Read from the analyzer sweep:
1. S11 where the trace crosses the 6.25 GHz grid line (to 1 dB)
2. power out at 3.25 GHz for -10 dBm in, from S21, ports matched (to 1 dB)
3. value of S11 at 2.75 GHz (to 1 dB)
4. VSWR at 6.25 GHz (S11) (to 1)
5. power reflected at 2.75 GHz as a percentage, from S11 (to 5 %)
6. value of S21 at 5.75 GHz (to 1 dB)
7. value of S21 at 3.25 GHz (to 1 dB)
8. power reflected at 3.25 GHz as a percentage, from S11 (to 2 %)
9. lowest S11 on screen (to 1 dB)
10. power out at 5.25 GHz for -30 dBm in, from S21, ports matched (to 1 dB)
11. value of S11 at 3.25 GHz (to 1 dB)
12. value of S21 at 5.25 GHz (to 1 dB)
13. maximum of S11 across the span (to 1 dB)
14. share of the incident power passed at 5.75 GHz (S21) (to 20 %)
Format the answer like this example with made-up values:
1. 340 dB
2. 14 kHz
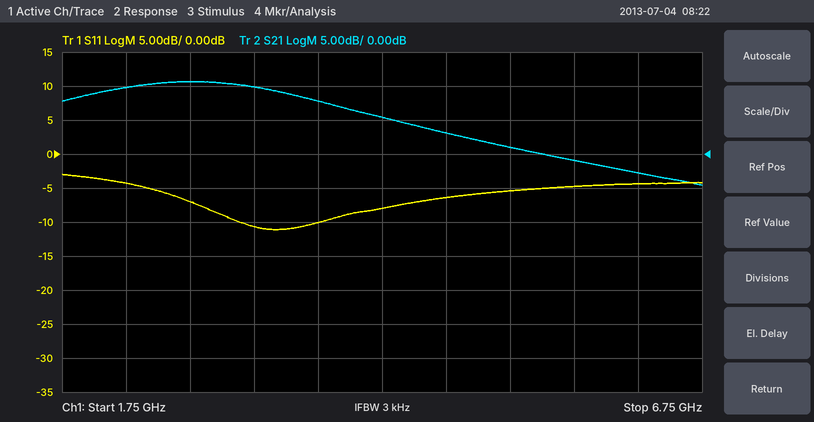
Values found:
1. -4 dB
2. 0 dBm
3. -7 dB
4. 4
5. 20 %
6. -1 dB
7. 10 dB
8. 8 %
9. -11 dB
10. -29 dBm
11. -11 dB
12. 1 dB
13. -3 dB
14. 80 %
